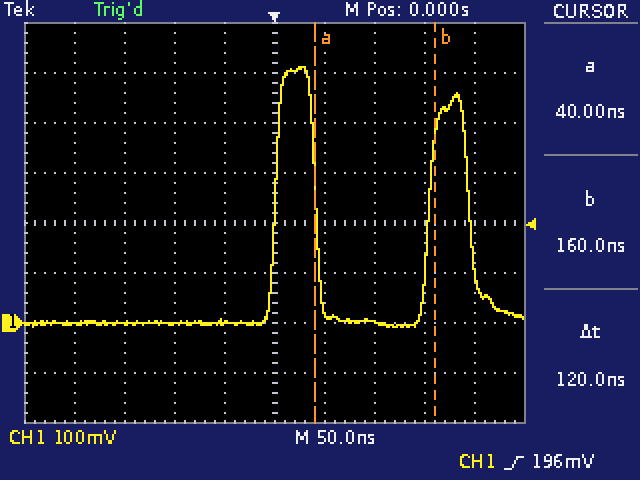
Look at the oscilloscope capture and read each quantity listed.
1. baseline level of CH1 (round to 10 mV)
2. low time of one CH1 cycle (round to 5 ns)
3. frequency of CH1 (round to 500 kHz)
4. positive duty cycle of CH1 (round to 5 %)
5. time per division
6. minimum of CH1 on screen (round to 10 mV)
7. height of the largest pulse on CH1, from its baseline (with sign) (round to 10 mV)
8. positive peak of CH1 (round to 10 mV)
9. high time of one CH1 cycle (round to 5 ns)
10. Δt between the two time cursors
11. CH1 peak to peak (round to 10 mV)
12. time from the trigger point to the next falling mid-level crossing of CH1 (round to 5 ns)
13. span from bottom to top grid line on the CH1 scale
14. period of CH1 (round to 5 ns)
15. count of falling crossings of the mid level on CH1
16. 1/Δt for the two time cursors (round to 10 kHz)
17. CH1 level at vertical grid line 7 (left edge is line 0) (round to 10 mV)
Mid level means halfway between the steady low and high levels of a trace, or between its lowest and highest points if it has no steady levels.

0 mV
115 ns
6.5 MHz
25 %
50 ns
-10 mV
+510 mV
510 mV
40 ns
120 ns
520 mV
40 ns
800 mV
155 ns
2
8.33 MHz
0 mV
